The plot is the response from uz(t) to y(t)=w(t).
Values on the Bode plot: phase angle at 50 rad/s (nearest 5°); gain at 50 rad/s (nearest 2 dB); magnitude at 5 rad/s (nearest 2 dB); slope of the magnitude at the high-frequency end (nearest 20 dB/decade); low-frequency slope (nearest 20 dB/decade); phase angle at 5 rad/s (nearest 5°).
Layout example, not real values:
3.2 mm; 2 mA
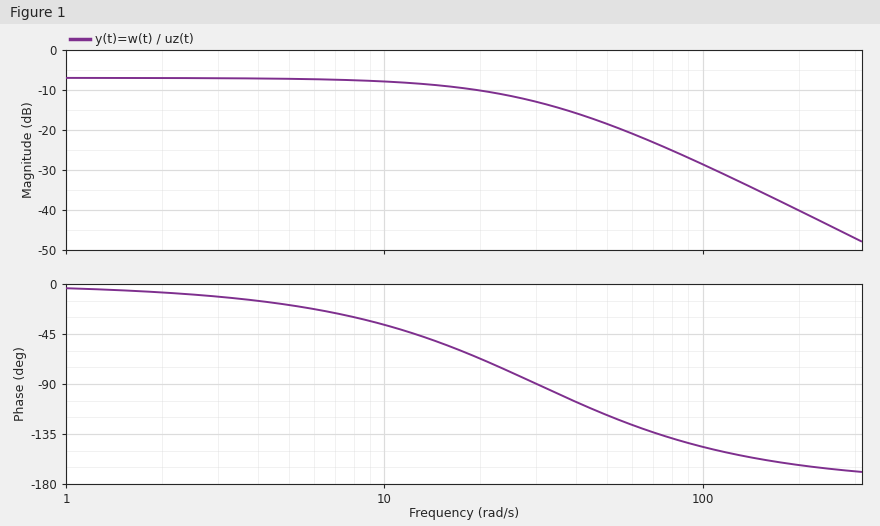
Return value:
-120°; -18 dB; -8 dB; -40 dB/decade; 0 dB/decade; -20°
